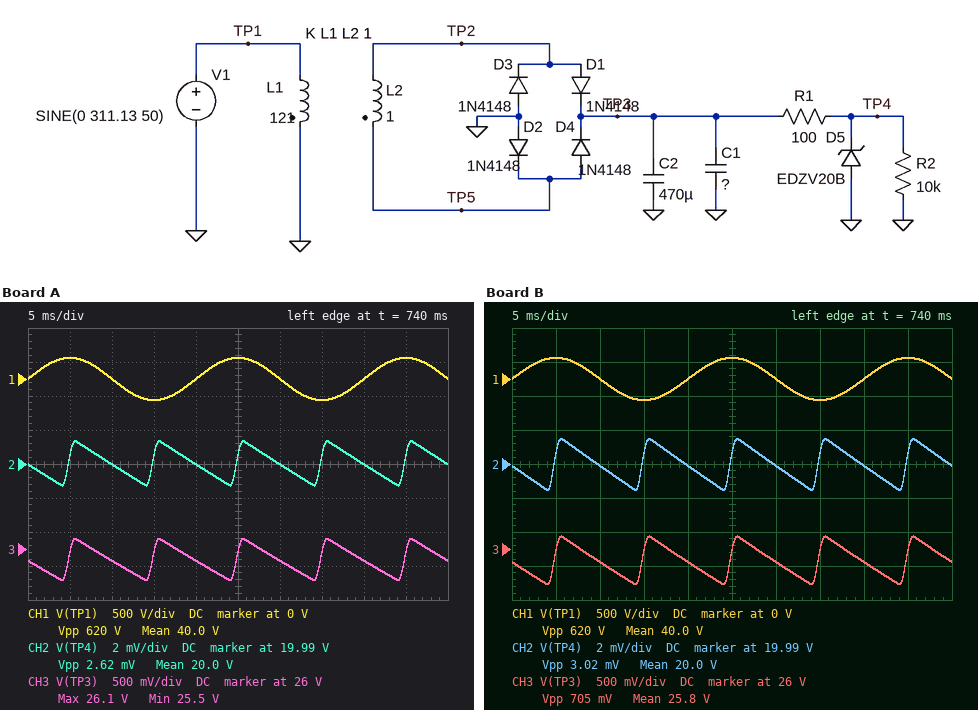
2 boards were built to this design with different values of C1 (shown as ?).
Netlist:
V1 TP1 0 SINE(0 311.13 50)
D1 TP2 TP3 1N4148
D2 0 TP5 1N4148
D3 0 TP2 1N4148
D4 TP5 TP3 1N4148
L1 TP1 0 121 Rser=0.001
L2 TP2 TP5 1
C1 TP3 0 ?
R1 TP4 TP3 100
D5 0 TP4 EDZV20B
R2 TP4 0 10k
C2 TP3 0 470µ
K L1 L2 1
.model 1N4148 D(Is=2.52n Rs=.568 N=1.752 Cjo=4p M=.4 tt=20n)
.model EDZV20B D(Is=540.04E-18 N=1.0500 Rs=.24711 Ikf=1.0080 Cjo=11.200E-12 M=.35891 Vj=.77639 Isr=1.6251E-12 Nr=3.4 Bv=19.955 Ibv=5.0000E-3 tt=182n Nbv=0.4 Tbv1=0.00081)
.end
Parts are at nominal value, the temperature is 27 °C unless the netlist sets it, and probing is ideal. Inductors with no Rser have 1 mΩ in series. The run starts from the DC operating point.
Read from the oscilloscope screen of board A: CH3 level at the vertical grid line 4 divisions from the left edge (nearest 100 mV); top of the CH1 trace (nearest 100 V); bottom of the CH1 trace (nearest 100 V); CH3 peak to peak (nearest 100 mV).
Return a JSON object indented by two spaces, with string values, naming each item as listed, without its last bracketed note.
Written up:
{
  "CH3 level at the vertical grid line 4 divisions from the left edge": "25.8 V",
  "top of the CH1 trace": "300 V",
  "bottom of the CH1 trace": "-300 V",
  "CH3 peak to peak": "600 mV"
}
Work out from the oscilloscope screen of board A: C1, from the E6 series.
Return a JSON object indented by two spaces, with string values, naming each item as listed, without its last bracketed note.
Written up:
{
  "C1, from the E6 series": "330 µF"
}
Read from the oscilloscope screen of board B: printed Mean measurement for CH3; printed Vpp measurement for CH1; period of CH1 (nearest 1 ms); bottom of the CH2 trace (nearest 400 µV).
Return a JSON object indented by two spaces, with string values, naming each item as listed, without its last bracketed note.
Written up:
{
  "printed Mean measurement for CH3": "25.8 V",
  "printed Vpp measurement for CH1": "620 V",
  "period of CH1": "20 ms",
  "bottom of the CH2 trace": "19.9924 V"
}
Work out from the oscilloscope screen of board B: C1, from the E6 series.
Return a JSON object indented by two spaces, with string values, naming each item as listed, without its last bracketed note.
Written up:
{
  "C1, from the E6 series": "220 µF"
}
